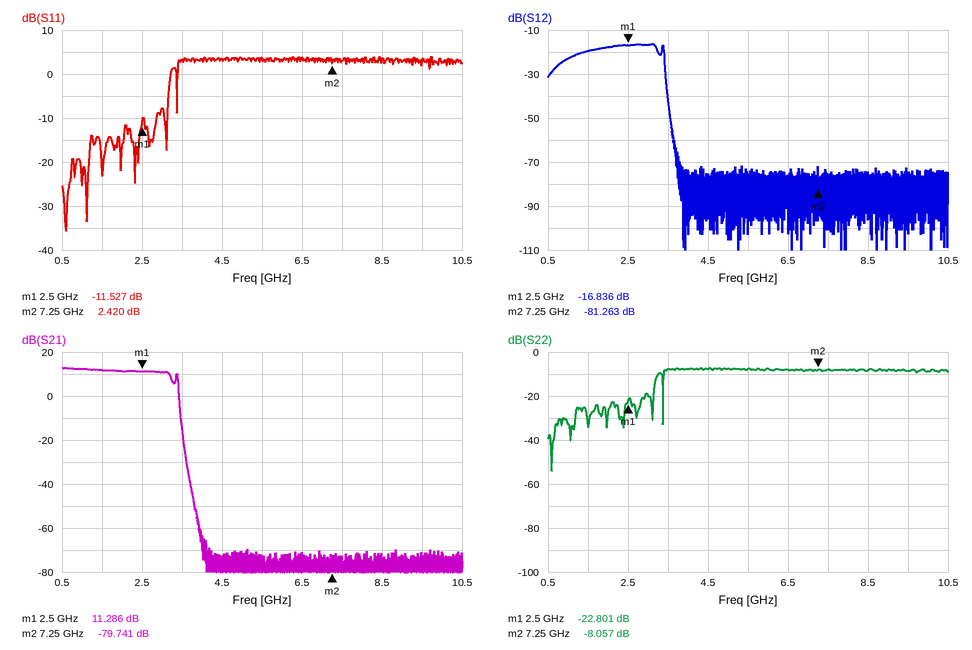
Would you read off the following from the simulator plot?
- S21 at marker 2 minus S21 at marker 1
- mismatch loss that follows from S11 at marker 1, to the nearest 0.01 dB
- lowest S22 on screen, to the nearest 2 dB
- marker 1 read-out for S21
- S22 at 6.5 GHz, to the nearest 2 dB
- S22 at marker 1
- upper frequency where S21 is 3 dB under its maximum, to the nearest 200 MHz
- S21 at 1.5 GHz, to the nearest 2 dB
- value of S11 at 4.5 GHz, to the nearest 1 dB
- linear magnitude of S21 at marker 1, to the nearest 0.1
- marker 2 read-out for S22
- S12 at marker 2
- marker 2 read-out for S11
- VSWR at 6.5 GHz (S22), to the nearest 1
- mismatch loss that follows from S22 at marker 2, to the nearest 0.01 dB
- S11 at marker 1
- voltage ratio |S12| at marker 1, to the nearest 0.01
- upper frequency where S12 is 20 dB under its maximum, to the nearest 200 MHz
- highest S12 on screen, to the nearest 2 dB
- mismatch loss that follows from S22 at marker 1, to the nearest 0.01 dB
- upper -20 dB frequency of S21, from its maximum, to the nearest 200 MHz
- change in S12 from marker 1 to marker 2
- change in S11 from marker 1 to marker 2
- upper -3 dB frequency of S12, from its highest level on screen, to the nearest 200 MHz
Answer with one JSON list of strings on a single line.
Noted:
["-91.027 dB", "0.32 dB", "-54 dB", "11.286 dB", "-8 dB", "-22.801 dB", "3.2 GHz", "12 dB", "3 dB", "3.7", "-8.057 dB", "-81.263 dB", "2.420 dB", "2", "0.74 dB", "-11.527 dB", "0.14", "3.4 GHz", "-16 dB", "0.02 dB", "3.4 GHz", "-64.427 dB", "13.947 dB", "3.2 GHz"]
